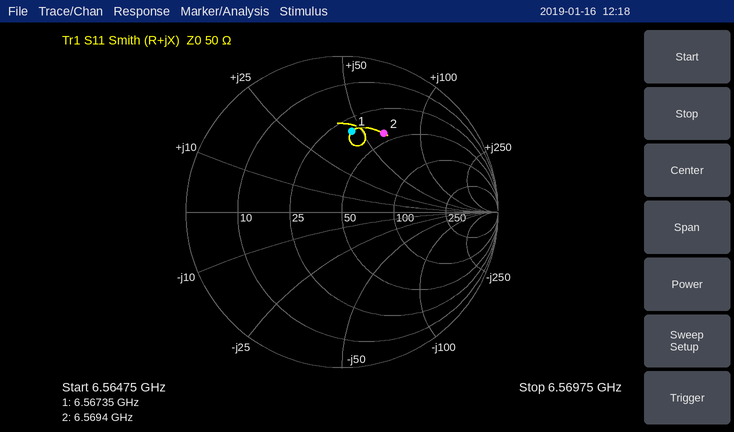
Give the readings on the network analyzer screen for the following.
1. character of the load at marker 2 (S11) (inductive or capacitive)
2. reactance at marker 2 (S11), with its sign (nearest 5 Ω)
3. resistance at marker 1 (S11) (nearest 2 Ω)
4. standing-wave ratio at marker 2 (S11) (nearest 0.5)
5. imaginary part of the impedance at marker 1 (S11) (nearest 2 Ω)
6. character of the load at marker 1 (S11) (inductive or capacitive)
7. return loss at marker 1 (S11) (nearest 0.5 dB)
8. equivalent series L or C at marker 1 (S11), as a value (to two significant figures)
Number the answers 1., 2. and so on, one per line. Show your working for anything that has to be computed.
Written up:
1. inductive
2. +65 Ω
3. 32 Ω
4. 3.5
5. +46 Ω
6. inductive
7. 5.5 dB
8. L = 46 Ω/(2π × 6.56735 GHz) ≈ 1.1 nH
